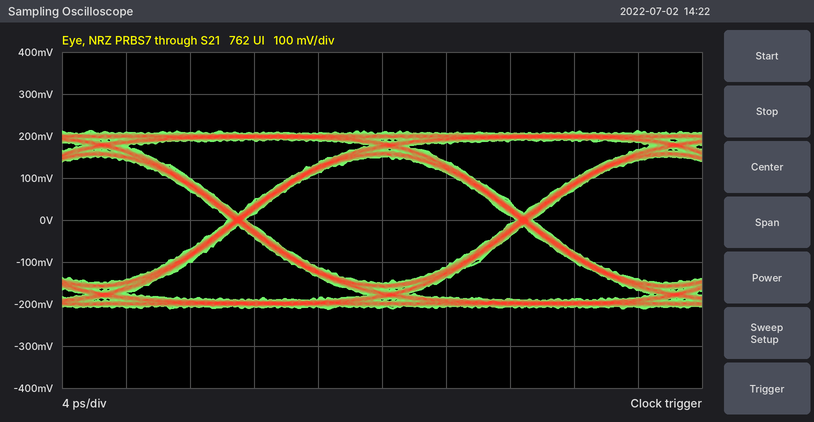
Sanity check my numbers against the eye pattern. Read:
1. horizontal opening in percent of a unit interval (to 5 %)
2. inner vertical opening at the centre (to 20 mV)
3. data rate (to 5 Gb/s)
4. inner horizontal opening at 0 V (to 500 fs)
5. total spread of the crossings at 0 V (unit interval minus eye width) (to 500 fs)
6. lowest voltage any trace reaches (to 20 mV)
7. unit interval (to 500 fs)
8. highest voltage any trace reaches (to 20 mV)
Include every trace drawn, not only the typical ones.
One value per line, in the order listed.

95 %
300 mV
55 Gb/s
17.0 ps
1.0 ps
-220 mV
18.0 ps
220 mV
